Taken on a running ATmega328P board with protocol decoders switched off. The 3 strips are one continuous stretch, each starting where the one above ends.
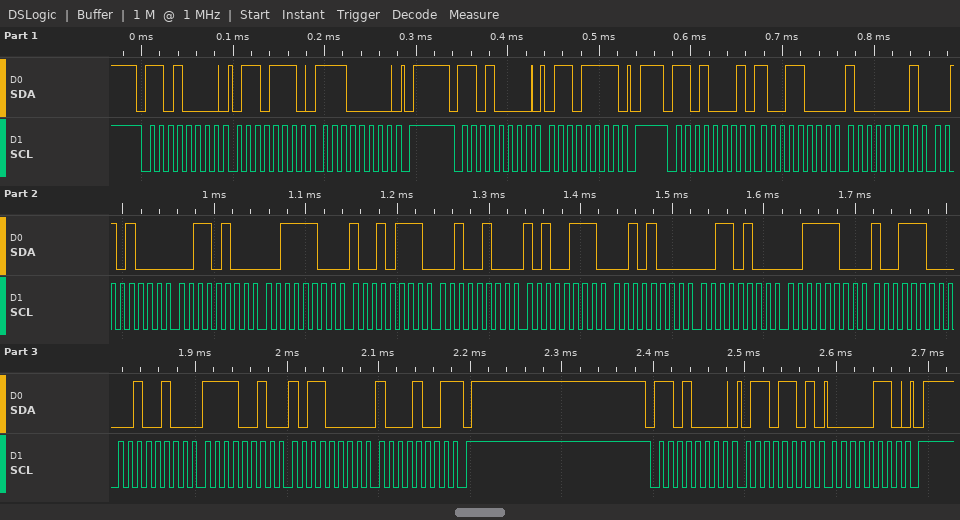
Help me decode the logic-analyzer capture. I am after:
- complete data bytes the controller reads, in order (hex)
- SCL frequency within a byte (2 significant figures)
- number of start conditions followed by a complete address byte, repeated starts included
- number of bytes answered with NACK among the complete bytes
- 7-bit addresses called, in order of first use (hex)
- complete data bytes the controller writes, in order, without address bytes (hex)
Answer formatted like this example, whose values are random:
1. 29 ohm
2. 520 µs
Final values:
1. 98 81 28 34 3C 97 24 A7 28 34 3C 9C 24 F2 B0 89
2. 100 kHz
3. 4
4. 1
5. 0x68
6. 6E E0 6F 6D 06
